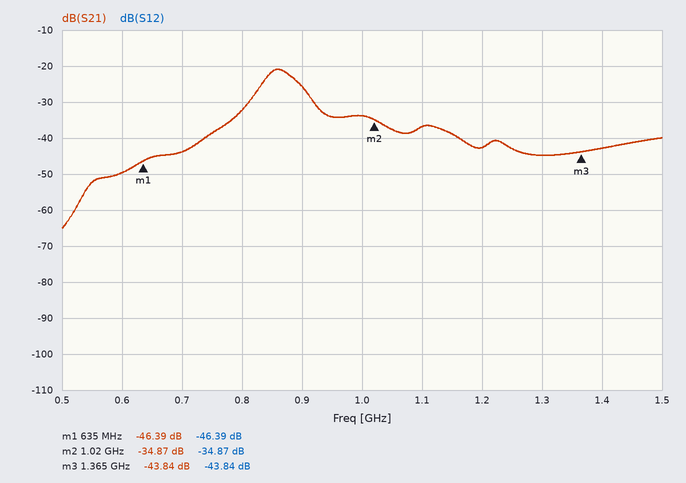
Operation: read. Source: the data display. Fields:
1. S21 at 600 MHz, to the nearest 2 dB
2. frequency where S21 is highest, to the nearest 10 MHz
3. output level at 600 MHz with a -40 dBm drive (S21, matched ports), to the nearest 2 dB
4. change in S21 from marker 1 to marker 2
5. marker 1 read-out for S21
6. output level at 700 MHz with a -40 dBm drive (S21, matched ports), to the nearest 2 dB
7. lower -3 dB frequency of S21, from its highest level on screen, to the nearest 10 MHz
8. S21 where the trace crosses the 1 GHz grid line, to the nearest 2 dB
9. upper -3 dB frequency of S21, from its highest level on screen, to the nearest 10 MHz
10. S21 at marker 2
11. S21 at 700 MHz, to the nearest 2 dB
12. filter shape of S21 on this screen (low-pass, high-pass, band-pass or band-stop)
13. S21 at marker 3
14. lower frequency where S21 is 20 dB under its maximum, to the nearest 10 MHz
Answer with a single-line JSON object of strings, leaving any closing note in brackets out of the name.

{"S21 at 600 MHz, to the nearest 2 dB": "-50 dB", "frequency where S21 is highest, to the nearest 10 MHz": "860 MHz", "output level at 600 MHz with a -40 dBm drive (S21, matched ports), to the nearest 2 dB": "-90 dBm", "change in S21 from marker 1 to marker 2": "11.52 dB", "marker 1 read-out for S21": "-46.39 dB", "output level at 700 MHz with a -40 dBm drive (S21, matched ports), to the nearest 2 dB": "-84 dBm", "lower -3 dB frequency of S21, from its highest level on screen, to the nearest 10 MHz": "840 MHz", "S21 where the trace crosses the 1 GHz grid line, to the nearest 2 dB": "-34 dB", "upper -3 dB frequency of S21, from its highest level on screen, to the nearest 10 MHz": "890 MHz", "S21 at marker 2": "-34.87 dB", "S21 at 700 MHz, to the nearest 2 dB": "-44 dB", "filter shape of S21 on this screen": "band-pass", "S21 at marker 3": "-43.84 dB", "lower frequency where S21 is 20 dB under its maximum, to the nearest 10 MHz": "730 MHz"}
